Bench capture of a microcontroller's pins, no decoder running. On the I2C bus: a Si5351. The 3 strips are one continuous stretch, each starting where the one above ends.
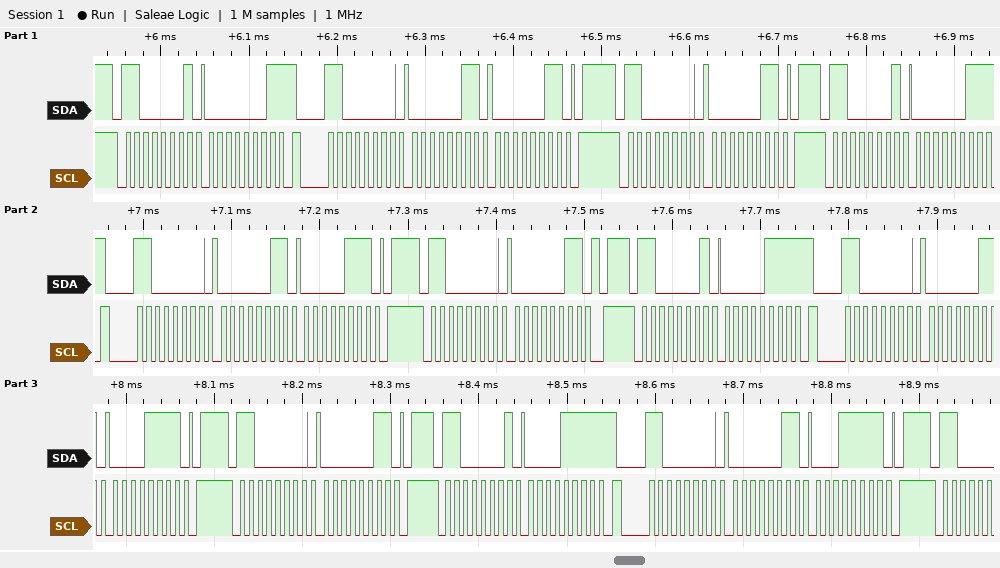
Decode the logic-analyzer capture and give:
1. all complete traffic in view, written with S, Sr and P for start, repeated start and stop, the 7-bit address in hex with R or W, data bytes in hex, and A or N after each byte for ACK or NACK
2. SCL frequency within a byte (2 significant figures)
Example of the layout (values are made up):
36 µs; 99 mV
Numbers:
S 60R A 01 N Sr 60W A 03 A 03 A P S 60W A 03 A P S 60R A 03 N Sr 60W A 03 A 07 A P S 60W A 03 A P S 60R A 07 N Sr 60W A 03 A 0F A P S 60W A 03 A P S 60R A 0F N Sr 60W A 03 A 1F A P; 100 kHz
